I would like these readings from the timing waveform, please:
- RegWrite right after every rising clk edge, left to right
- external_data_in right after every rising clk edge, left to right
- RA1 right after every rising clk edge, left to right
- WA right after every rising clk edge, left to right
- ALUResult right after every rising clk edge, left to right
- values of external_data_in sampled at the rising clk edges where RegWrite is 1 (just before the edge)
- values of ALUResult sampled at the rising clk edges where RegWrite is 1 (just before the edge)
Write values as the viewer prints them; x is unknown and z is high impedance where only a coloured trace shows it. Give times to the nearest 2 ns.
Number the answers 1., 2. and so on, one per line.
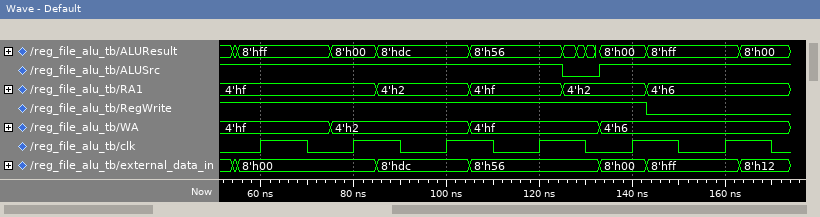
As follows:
1. 1 1 1 1 1 0
2. 8'h00, 8'h00, 8'hdc, 8'h56, 8'h00, 8'hff
3. 4'hf, 4'hf, 4'h2, 4'hf, 4'h2, 4'h6
4. 4'hf, 4'h2, 4'h2, 4'hf, 4'h6, 4'h6
5. 8'hff, 8'h00, 8'hdc, 8'h56, 8'h00, 8'hff
6. 8'h00, 8'h00, 8'hdc, 8'h56, 8'h00
7. 8'hff, 8'h00, 8'hdc, 8'h56, 8'h00
